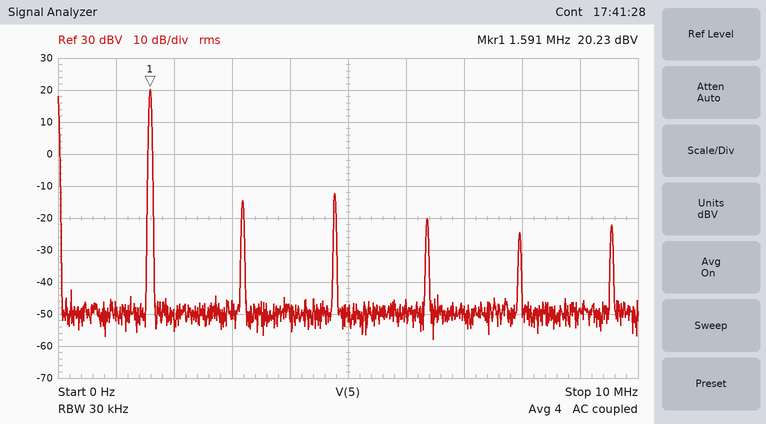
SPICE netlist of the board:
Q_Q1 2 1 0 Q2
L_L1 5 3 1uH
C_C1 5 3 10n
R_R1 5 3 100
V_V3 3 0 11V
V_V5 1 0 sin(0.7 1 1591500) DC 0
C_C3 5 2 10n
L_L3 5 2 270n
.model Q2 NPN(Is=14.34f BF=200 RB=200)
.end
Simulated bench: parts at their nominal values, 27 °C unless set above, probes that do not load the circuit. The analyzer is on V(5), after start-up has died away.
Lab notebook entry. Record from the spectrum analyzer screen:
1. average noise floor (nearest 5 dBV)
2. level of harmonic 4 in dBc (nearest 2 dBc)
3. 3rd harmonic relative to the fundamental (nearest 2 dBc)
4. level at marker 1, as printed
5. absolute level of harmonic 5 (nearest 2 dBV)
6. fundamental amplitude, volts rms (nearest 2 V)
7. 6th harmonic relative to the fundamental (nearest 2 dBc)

-50 dBV
-40 dBc
-32 dBc
20.23 dBV
-24 dBV
10 V
-42 dBc
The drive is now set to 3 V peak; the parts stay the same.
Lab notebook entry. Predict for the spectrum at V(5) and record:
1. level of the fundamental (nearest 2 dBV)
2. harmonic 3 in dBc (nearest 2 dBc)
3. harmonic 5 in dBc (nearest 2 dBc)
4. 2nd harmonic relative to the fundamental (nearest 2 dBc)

22 dBV
-34 dBc
-36 dBc
-30 dBc
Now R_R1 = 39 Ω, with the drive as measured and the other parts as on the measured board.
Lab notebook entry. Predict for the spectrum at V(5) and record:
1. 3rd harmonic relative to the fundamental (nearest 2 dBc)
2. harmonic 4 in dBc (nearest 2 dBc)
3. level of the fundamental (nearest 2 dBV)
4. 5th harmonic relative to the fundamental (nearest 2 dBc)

-28 dBc
-30 dBc
18 dBV
-36 dBc
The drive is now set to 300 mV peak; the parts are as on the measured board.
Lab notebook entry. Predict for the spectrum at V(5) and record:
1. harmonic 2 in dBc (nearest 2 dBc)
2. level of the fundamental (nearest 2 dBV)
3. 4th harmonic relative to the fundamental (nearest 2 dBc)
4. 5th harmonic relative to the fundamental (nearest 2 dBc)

-30 dBc
16 dBV
-50 dBc
-56 dBc
